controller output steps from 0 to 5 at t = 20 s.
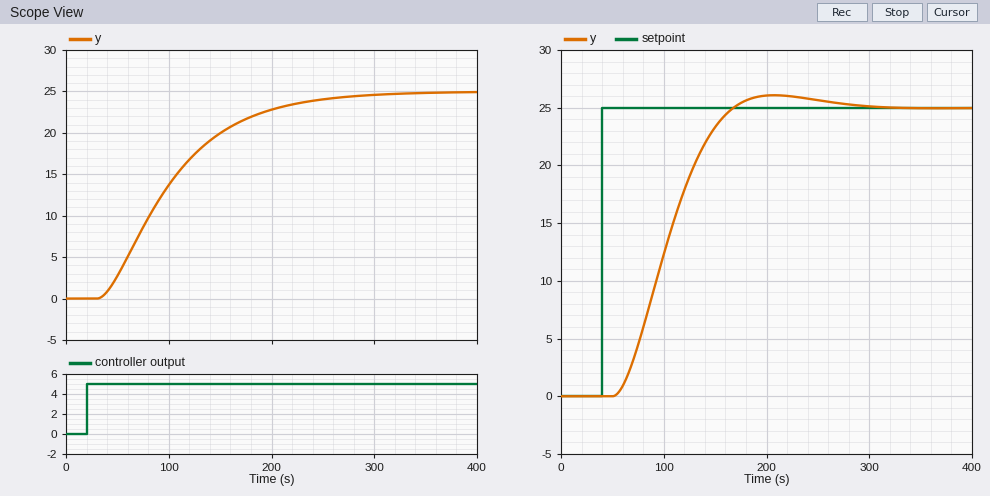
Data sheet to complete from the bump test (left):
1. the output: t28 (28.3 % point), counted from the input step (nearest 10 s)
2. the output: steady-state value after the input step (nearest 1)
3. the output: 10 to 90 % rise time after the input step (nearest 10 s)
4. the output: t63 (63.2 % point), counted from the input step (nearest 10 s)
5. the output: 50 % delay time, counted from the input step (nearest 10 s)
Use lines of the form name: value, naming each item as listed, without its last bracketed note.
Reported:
the output: t28 (28.3 % point), counted from the input step: 50 s
the output: steady-state value after the input step: 25
the output: 10 to 90 % rise time after the input step: 140 s
the output: t63 (63.2 % point), counted from the input step: 90 s
the output: 50 % delay time, counted from the input step: 70 s
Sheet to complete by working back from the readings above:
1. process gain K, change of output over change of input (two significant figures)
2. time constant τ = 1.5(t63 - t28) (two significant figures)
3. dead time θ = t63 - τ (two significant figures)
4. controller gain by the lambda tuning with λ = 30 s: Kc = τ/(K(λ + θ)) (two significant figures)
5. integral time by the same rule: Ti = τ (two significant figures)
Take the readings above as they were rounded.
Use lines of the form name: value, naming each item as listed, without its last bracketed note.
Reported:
process gain K, change of output over change of input: 5.0
time constant τ = 1.5(t63 - t28): 60 s
dead time θ = t63 - τ: 30 s
controller gain by the lambda tuning with λ = 30 s: Kc = τ/(K(λ + θ)): 0.20
integral time by the same rule: Ti = τ: 60 s
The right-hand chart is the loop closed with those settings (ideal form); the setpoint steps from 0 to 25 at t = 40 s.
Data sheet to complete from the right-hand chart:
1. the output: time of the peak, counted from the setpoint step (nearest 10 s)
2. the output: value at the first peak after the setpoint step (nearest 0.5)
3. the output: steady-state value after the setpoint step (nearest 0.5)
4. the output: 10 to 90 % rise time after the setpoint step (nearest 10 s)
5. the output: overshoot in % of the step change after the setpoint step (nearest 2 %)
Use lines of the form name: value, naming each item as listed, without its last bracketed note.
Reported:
the output: time of the peak, counted from the setpoint step: 170 s
the output: value at the first peak after the setpoint step: 26.0
the output: steady-state value after the setpoint step: 25.0
the output: 10 to 90 % rise time after the setpoint step: 80 s
the output: overshoot in % of the step change after the setpoint step: 4 %
